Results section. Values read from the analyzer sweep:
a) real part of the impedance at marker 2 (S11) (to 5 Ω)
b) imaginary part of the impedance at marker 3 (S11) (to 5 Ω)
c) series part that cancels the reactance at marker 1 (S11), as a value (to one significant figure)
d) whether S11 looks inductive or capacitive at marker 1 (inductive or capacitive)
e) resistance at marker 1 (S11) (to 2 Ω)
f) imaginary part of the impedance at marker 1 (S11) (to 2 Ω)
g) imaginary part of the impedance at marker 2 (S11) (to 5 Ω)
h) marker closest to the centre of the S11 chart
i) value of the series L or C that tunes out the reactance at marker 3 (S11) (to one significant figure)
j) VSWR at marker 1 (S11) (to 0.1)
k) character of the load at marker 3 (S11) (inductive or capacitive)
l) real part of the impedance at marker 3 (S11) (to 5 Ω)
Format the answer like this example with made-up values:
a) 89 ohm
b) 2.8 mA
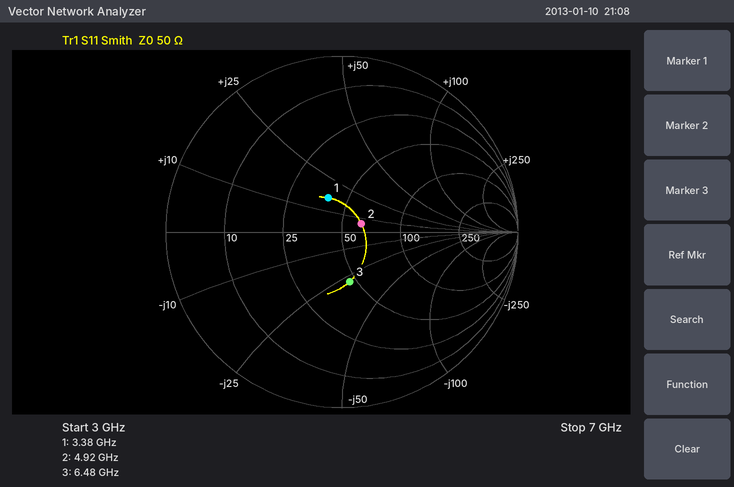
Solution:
a) 60 Ω
b) -30 Ω
c) 3 pF
d) inductive
e) 40 Ω
f) +16 Ω
g) +5 Ω
h) marker 2
i) 700 pH
j) 1.5
k) capacitive
l) 45 Ω
